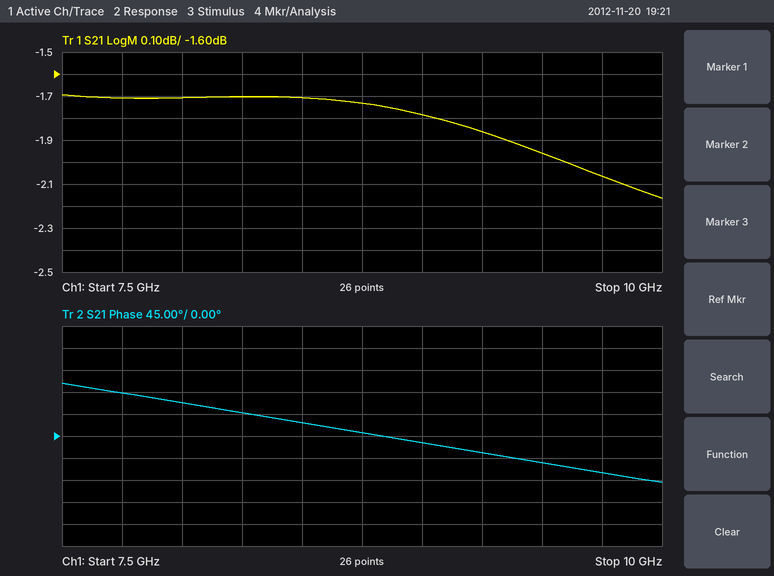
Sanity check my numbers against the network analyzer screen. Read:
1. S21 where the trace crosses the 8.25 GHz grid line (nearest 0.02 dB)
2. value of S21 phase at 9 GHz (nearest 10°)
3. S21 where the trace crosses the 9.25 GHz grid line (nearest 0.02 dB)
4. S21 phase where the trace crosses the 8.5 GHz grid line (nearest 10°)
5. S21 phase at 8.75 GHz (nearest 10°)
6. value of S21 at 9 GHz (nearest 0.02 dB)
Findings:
-1.70 dB
-10°
-1.86 dB
30°
10°
-1.78 dB
